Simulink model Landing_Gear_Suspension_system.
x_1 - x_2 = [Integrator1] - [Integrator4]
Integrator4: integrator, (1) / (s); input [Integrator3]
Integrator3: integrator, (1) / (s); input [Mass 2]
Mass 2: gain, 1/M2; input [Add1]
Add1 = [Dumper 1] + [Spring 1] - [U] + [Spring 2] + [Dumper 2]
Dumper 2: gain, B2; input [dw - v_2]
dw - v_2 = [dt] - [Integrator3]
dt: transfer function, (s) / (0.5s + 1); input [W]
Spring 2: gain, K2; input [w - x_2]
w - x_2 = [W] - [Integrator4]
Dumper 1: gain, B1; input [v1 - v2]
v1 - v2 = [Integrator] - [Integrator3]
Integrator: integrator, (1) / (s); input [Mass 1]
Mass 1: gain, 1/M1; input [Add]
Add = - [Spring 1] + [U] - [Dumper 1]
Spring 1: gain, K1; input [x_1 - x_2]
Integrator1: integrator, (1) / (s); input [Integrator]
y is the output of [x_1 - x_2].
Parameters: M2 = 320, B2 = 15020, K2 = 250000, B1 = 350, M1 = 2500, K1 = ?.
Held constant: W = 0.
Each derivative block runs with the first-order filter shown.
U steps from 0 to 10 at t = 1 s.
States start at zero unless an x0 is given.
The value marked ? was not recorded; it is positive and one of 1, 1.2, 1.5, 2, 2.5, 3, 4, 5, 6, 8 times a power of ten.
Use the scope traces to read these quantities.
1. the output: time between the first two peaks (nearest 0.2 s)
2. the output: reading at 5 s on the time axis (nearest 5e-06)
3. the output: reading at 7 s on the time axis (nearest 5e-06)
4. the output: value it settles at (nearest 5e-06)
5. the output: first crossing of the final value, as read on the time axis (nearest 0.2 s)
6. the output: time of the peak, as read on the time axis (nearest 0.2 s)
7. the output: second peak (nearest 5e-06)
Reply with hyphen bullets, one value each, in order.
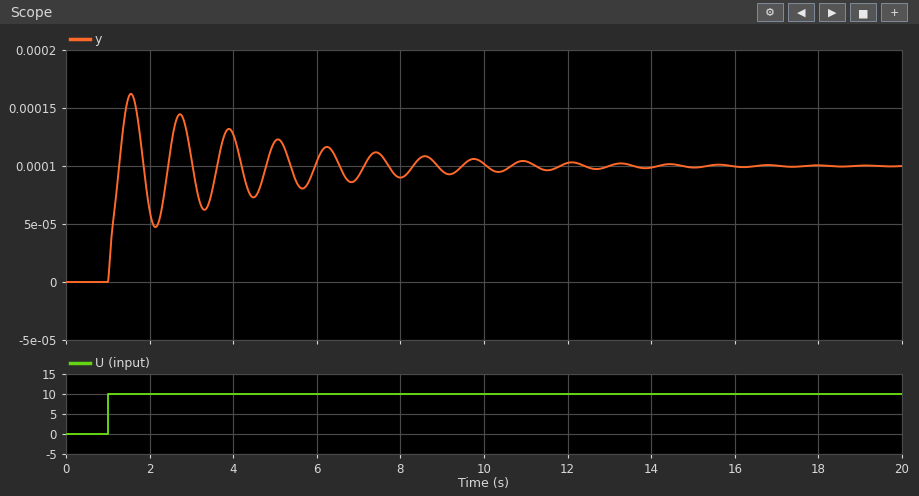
- 1.2 s
- 0.000120
- 0.000090
- 0.000100
- 1.2 s
- 1.6 s
- 0.000145
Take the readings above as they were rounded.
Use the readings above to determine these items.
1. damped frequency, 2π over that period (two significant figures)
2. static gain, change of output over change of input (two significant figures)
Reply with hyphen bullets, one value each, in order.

- 5.2 rad/s
- 0.000010
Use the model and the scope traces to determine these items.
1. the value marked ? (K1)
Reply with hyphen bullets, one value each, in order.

- 100000
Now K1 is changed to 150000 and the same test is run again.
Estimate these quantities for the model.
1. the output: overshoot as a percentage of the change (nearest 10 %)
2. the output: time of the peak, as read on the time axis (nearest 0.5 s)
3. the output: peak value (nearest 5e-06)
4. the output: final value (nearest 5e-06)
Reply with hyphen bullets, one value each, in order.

- 50 %
- 1.5 s
- 0.000100
- 0.000065
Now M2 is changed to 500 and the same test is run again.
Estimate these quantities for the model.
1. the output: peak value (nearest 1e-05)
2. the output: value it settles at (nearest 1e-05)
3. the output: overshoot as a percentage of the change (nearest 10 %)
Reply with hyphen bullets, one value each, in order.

- 0.00016
- 0.00010
- 60 %
